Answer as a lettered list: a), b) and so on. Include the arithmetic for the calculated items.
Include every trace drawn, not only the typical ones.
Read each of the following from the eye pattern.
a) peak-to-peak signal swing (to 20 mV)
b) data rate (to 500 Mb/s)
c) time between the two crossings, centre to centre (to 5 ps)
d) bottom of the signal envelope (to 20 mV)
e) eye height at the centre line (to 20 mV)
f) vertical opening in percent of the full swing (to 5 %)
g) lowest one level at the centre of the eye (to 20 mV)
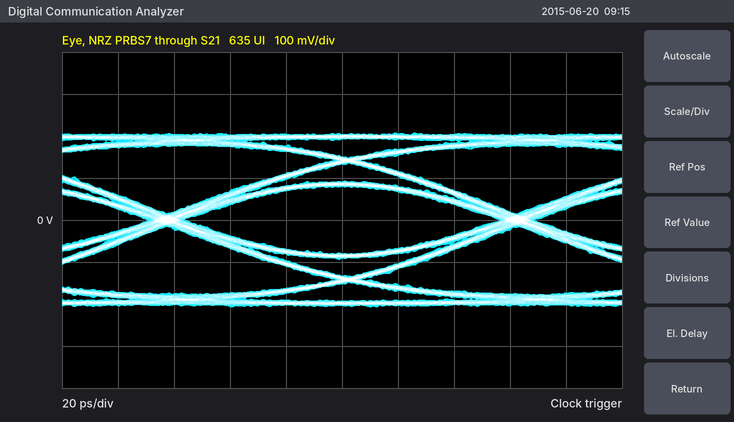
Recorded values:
a) 420 mV
b) 8.0 Gb/s
c) 125 ps
d) -200 mV
e) 160 mV
f) 160 mV / 420 mV ≈ 38.1 %, so 40 % to the nearest 5 %
g) 80 mV
